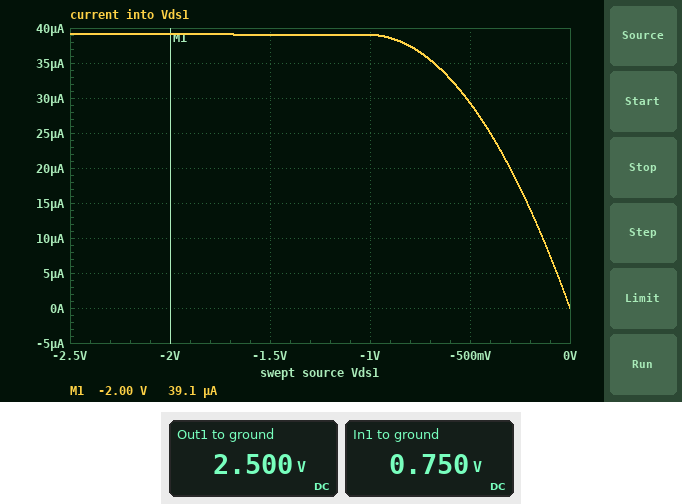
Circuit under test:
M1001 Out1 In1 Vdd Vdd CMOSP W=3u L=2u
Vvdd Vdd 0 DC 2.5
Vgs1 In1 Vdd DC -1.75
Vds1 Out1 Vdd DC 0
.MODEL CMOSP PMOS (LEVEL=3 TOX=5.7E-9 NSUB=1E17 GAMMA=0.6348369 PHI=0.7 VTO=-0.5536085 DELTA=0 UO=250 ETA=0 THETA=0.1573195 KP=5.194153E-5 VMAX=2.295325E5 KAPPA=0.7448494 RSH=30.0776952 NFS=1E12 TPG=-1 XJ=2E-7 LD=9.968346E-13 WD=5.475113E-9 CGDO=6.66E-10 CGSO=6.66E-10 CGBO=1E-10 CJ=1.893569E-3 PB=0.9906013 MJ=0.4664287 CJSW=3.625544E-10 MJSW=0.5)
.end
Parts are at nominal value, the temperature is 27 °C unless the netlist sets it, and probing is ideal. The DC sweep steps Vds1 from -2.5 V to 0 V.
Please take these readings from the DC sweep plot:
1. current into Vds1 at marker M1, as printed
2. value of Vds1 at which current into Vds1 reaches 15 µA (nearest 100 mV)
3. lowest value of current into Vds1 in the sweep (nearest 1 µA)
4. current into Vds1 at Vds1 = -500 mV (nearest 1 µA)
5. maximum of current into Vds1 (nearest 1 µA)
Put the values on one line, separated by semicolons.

39.1 µA; -200 mV; 0 A; 29 µA; 39 µA
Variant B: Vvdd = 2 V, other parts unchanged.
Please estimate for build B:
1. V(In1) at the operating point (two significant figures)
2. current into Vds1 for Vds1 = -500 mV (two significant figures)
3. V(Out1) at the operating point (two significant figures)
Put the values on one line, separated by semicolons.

250 mV; 29 µA; 2.0 V
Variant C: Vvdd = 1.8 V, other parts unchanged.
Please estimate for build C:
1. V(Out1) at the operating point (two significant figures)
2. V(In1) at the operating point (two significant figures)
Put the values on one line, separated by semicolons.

1.8 V; 50 mV
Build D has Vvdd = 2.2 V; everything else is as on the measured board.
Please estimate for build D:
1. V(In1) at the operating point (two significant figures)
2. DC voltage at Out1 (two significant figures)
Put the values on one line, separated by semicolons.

450 mV; 2.2 V
